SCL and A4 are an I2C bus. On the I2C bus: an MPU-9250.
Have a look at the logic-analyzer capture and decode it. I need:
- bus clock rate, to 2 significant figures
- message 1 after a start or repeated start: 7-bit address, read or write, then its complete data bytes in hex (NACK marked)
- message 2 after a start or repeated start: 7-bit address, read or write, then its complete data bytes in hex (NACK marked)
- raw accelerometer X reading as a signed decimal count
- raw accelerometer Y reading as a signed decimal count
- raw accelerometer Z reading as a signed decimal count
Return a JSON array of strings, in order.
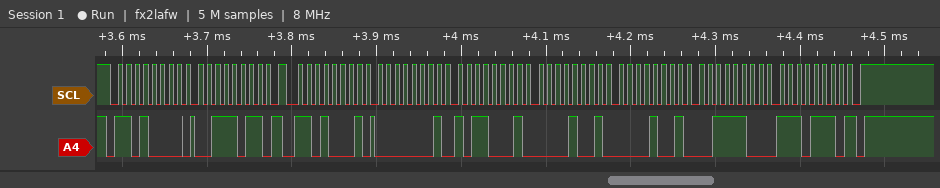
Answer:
["100 kHz", "0x68 write: 3B", "0x68 read: 01 B1 09 09 3C EE NACK", "433", "2313", "15598"]
